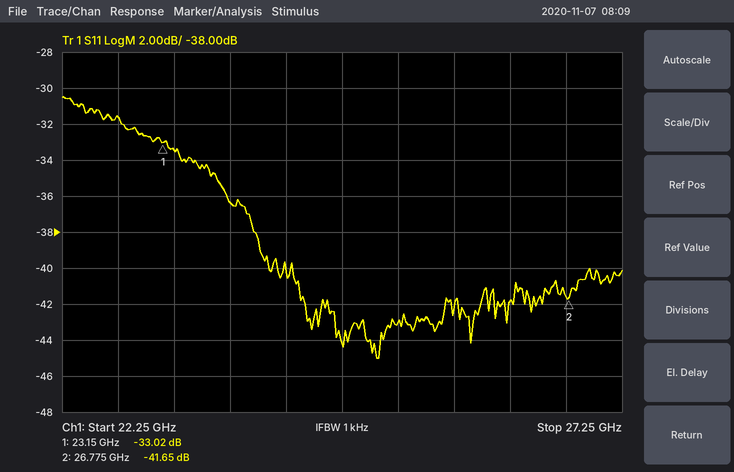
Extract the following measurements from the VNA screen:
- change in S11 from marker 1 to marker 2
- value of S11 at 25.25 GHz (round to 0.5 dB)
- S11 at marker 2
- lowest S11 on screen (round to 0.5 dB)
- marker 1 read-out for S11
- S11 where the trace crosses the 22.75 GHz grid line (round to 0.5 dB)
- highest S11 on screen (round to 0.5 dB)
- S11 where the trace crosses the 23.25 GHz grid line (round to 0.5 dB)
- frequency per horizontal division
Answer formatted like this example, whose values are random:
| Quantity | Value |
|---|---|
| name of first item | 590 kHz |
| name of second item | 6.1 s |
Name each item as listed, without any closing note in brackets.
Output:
| Quantity | Value |
|---|---|
| change in S11 from marker 1 to marker 2 | -8.63 dB |
| value of S11 at 25.25 GHz | -43.0 dB |
| S11 at marker 2 | -41.65 dB |
| lowest S11 on screen | -45.0 dB |
| marker 1 read-out for S11 | -33.02 dB |
| S11 where the trace crosses the 22.75 GHz grid line | -31.5 dB |
| highest S11 on screen | -30.5 dB |
| S11 where the trace crosses the 23.25 GHz grid line | -33.5 dB |
| frequency per horizontal division | 500 MHz |
